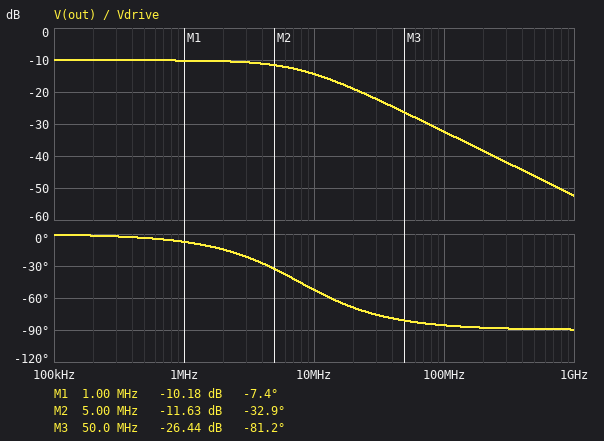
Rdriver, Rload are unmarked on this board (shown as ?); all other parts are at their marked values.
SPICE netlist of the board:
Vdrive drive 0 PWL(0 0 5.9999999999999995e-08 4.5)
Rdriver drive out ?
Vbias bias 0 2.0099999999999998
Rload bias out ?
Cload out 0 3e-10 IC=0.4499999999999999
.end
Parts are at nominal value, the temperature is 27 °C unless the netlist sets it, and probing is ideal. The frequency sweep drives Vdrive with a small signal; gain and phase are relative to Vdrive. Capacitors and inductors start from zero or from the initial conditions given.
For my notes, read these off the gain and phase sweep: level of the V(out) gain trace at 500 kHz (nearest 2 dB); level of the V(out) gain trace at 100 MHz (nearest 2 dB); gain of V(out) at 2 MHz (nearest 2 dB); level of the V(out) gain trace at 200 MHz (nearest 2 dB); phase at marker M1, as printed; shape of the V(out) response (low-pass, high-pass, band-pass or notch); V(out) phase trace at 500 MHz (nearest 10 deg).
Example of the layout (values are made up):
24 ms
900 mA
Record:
-10 dB
-32 dB
-10 dB
-38 dB
-7.4 deg
low-pass
-90 deg
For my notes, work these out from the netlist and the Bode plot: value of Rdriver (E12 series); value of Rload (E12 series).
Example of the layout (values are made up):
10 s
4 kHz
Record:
220 Ω
100 Ω
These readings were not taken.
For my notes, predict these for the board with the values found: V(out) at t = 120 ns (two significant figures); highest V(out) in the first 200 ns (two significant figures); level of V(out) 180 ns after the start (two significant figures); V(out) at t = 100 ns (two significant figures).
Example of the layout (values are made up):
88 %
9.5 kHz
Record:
2.8 V
2.8 V
2.8 V
2.7 V
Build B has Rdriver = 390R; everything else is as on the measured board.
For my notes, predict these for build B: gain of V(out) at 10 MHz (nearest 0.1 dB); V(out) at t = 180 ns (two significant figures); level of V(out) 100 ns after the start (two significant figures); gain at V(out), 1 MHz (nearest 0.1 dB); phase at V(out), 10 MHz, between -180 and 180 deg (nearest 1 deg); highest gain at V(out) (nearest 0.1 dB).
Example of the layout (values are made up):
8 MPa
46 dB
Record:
-18.9 dB
2.5 V
2.4 V
-13.9 dB
-56 deg
-13.8 dB
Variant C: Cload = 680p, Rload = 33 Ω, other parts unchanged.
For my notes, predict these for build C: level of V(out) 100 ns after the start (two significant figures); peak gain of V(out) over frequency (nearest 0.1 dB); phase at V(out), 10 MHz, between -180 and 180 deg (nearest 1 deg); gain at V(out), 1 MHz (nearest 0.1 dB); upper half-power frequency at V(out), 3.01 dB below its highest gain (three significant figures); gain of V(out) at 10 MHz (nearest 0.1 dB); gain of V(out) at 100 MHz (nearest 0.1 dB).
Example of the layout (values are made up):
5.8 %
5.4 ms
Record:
2.3 V
-17.7 dB
-51 deg
-17.8 dB
8.16 MHz
-21.7 dB
-39.5 dB
